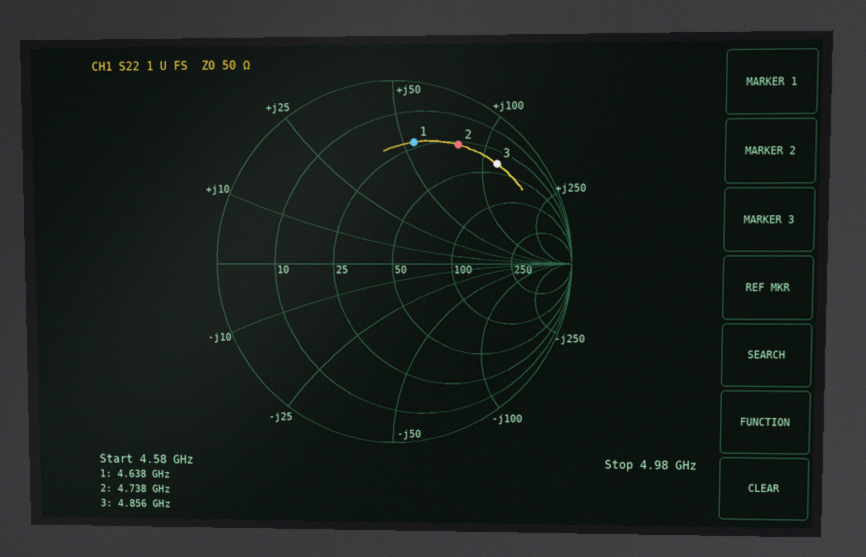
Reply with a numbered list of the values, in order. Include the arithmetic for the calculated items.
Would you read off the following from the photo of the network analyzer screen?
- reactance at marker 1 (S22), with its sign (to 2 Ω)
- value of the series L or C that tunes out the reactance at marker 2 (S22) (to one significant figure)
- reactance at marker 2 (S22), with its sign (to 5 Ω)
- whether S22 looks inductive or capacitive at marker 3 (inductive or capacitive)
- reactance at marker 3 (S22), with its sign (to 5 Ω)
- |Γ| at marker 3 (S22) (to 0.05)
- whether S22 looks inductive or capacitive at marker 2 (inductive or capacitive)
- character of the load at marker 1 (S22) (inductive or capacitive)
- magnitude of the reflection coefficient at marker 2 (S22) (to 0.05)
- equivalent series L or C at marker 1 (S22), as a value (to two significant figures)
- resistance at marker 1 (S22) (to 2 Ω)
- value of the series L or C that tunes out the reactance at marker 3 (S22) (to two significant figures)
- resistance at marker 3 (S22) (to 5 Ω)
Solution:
1. +54 Ω
2. C = 1/(2π × 4.738 GHz × 80 Ω) ≈ 420 fF, so 400 fF to one significant figure
3. +80 Ω
4. inductive
5. +115 Ω
6. 0.80
7. inductive
8. inductive
9. 0.75
10. L = 54 Ω/(2π × 4.638 GHz) ≈ 1.9 nH
11. 22 Ω
12. C = 1/(2π × 4.856 GHz × 115 Ω) ≈ 285 fF, so 280 fF to two significant figures
13. 40 Ω
